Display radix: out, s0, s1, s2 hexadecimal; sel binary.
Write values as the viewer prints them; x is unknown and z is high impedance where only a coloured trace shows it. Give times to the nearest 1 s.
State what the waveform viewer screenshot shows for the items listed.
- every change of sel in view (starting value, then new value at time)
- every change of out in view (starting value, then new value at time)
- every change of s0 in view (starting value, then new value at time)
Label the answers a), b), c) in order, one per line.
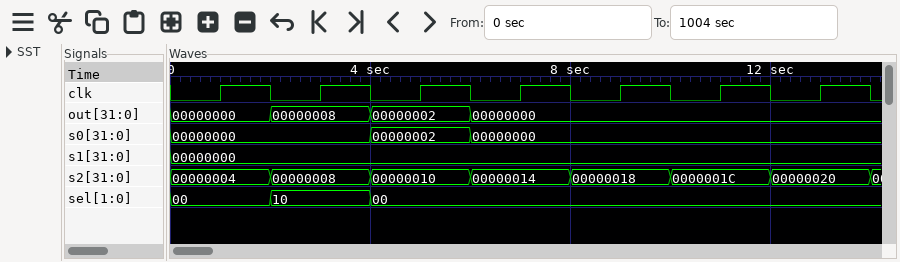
a) 00, 10 at 2 s, 00 at 4 s
b) 00000000, 00000008 at 2 s, 00000002 at 4 s, 00000000 at 6 s
c) 00000000, 00000002 at 4 s, 00000000 at 6 s
